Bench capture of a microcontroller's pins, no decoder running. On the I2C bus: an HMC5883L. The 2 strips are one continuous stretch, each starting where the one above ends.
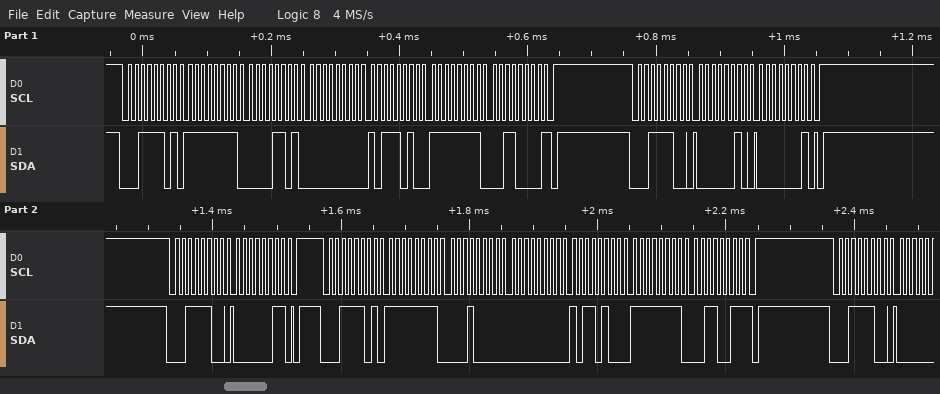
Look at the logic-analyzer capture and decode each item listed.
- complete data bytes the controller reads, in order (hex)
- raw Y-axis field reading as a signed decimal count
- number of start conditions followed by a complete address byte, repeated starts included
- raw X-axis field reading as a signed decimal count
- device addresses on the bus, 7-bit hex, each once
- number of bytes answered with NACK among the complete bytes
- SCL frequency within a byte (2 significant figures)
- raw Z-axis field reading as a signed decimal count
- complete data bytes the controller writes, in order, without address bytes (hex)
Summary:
FF 0D 00 BA FF 30 FF 10 00 B4 FF 33
-205
5
-240
0x1E
2
100 kHz
180
02 01 03
